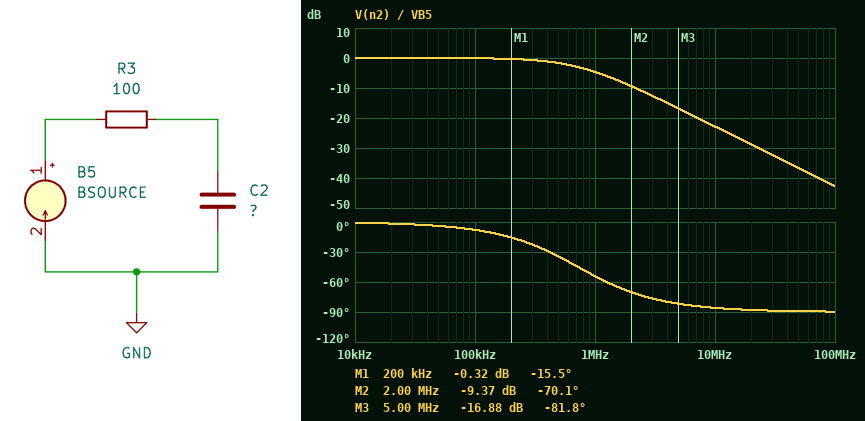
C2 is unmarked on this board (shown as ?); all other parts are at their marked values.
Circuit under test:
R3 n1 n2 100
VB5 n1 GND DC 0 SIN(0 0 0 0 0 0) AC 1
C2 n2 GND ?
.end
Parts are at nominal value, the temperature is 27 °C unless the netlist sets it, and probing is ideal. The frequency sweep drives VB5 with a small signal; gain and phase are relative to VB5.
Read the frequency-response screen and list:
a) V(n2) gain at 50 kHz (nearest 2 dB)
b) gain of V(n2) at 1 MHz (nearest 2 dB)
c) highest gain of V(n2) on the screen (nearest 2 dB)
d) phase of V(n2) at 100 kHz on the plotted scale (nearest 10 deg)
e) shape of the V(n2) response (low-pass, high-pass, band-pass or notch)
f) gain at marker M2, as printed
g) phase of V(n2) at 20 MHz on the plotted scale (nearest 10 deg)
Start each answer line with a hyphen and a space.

- 0 dB
- -4 dB
- 0 dB
- -10 deg
- low-pass
- -9.37 dB
- -90 deg
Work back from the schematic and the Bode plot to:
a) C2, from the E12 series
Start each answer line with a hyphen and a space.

- 2.2 nF
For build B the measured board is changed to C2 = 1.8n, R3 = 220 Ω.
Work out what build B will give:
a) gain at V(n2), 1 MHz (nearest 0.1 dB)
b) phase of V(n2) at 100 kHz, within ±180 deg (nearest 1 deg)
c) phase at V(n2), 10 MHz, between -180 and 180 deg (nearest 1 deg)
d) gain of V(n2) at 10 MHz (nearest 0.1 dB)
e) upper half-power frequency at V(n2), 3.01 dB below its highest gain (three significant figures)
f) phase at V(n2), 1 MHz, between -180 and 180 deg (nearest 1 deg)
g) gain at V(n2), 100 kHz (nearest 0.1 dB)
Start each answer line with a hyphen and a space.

- -8.6 dB
- -14 deg
- -88 deg
- -27.9 dB
- 402 kHz
- -68 deg
- -0.3 dB
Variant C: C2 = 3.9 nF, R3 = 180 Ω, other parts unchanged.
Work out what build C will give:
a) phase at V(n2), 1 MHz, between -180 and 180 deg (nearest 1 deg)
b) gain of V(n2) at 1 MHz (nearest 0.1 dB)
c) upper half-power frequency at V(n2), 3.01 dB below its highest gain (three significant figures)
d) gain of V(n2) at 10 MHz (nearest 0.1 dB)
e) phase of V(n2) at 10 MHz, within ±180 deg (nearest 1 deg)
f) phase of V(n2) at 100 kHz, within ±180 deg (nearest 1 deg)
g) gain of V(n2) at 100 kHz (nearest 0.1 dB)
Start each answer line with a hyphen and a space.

- -77 deg
- -13.1 dB
- 227 kHz
- -32.9 dB
- -89 deg
- -24 deg
- -0.8 dB
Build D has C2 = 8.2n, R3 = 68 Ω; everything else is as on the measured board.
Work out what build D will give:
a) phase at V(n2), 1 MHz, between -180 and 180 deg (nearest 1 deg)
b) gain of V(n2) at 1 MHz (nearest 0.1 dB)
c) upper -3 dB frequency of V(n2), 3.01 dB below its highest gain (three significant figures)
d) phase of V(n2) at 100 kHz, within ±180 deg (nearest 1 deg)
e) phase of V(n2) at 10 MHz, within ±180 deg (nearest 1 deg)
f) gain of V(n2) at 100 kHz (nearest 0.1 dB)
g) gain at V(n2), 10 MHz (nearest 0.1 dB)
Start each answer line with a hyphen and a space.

- -74 deg
- -11.2 dB
- 285 kHz
- -19 deg
- -88 deg
- -0.5 dB
- -30.9 dB
